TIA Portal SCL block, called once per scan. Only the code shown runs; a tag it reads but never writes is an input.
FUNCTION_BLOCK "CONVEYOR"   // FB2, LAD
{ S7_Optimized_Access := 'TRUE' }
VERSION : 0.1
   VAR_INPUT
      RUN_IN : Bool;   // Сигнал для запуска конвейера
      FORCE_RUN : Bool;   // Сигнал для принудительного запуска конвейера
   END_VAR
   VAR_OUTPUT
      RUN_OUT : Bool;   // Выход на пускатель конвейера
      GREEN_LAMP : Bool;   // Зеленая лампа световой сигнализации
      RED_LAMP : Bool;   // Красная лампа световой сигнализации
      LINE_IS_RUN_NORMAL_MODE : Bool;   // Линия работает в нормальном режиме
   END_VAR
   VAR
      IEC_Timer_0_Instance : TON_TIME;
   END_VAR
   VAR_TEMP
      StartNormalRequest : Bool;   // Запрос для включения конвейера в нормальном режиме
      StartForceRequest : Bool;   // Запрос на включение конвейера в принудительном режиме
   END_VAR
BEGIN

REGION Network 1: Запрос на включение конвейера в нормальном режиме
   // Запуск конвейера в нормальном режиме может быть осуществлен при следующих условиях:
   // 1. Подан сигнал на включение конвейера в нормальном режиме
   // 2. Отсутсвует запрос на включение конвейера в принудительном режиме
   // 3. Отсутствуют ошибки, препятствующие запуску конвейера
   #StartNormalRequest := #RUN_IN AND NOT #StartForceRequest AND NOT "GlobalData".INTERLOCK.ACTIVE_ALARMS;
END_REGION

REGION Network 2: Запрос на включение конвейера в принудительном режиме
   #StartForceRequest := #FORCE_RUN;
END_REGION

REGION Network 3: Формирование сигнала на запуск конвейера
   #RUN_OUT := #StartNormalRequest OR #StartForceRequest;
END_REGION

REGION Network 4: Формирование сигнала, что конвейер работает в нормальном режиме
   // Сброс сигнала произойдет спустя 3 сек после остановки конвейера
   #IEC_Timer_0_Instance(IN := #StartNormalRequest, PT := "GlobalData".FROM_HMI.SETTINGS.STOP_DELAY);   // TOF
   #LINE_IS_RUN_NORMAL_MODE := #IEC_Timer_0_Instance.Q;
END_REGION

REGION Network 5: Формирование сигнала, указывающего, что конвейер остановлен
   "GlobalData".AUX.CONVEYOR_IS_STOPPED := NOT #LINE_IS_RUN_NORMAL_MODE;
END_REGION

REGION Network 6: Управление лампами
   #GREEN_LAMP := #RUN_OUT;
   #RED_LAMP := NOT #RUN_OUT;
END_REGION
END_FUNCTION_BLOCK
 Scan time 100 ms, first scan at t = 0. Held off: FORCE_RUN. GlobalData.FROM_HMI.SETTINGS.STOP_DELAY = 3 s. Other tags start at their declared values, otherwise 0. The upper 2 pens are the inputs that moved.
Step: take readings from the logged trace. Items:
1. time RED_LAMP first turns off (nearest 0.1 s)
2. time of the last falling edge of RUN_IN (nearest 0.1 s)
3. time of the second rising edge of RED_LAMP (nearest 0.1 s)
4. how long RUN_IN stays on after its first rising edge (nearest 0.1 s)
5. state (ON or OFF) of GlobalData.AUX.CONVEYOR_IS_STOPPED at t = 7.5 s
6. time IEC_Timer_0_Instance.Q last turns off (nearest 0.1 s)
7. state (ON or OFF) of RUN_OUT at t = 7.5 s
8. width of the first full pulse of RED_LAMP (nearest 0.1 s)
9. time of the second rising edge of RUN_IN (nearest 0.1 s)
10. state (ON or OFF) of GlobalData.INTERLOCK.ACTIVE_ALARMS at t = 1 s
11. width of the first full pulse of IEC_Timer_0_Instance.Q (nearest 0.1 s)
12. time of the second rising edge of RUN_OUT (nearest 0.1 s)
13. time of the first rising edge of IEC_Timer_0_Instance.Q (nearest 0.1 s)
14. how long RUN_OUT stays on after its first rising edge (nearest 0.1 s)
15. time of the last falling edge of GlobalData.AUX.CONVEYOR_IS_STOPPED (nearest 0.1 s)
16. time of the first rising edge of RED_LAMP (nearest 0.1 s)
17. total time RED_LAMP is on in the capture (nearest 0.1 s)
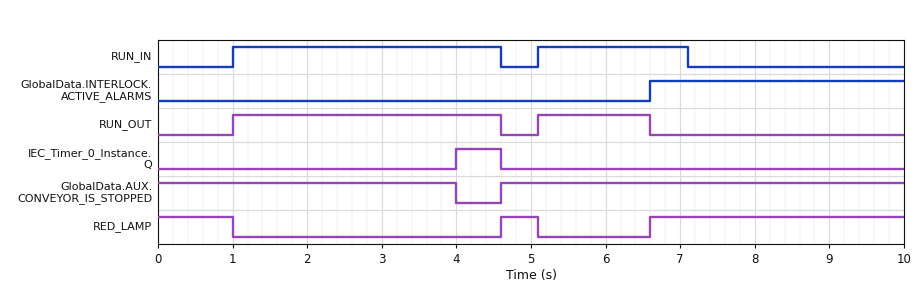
1.0 s
7.1 s
6.6 s
3.6 s
ON
4.6 s
OFF
0.5 s
5.1 s
OFF
0.6 s
5.1 s
4.0 s
3.6 s
4.0 s
4.6 s
4.9 s
